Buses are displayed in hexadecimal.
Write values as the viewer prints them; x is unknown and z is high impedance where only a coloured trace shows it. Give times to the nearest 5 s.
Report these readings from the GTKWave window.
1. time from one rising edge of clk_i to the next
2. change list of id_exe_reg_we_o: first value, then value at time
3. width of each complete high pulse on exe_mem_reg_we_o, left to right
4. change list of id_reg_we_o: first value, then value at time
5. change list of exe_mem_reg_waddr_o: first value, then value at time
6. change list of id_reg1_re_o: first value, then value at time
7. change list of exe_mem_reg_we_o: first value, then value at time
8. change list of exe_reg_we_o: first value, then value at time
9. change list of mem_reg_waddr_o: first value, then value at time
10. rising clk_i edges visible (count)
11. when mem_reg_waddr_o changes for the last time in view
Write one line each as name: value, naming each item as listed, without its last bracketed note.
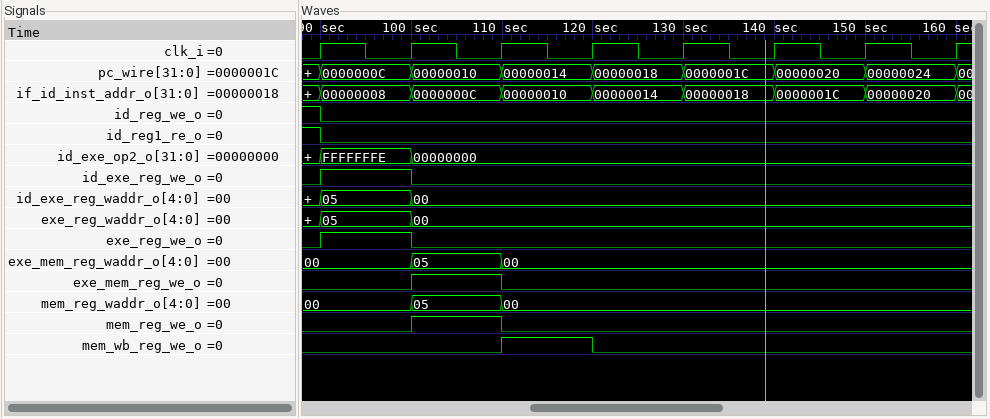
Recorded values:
time from one rising edge of clk_i to the next: 10 s
change list of id_exe_reg_we_o: first value, then value at time: 0, 1 at 90 s, 0 at 100 s
width of each complete high pulse on exe_mem_reg_we_o, left to right: 10 s
change list of id_reg_we_o: first value, then value at time: 1, 0 at 90 s
change list of exe_mem_reg_waddr_o: first value, then value at time: 00, 05 at 100 s, 00 at 110 s
change list of id_reg1_re_o: first value, then value at time: 1, 0 at 90 s
change list of exe_mem_reg_we_o: first value, then value at time: 0, 1 at 100 s, 0 at 110 s
change list of exe_reg_we_o: first value, then value at time: 0, 1 at 90 s, 0 at 100 s
change list of mem_reg_waddr_o: first value, then value at time: 00, 05 at 100 s, 00 at 110 s
rising clk_i edges visible: 8
when mem_reg_waddr_o changes for the last time in view: 110 s
